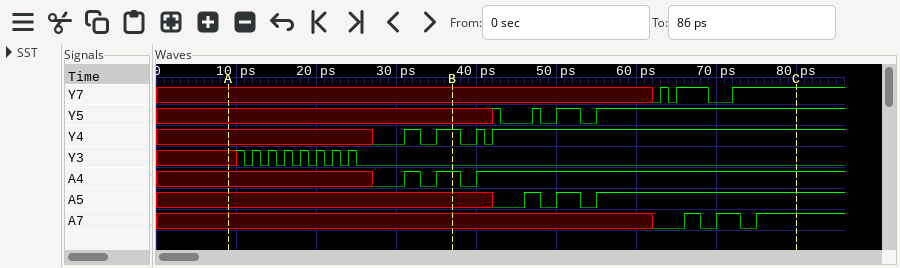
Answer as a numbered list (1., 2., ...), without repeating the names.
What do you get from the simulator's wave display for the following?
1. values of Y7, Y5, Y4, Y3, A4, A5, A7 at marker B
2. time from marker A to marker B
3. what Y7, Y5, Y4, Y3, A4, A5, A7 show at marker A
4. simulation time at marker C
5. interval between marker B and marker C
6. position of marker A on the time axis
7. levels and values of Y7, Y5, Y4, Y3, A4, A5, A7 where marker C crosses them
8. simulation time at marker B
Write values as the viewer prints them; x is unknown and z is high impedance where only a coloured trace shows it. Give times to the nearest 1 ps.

1. Y7=x, Y5=x, Y4=1, Y3=0, A4=1, A5=x, A7=x
2. 28 ps
3. Y7=x, Y5=x, Y4=x, Y3=x, A4=x, A5=x, A7=x
4. 80 ps
5. 43 ps
6. 9 ps
7. Y7=1, Y5=1, Y4=1, Y3=0, A4=1, A5=1, A7=1
8. 37 ps
